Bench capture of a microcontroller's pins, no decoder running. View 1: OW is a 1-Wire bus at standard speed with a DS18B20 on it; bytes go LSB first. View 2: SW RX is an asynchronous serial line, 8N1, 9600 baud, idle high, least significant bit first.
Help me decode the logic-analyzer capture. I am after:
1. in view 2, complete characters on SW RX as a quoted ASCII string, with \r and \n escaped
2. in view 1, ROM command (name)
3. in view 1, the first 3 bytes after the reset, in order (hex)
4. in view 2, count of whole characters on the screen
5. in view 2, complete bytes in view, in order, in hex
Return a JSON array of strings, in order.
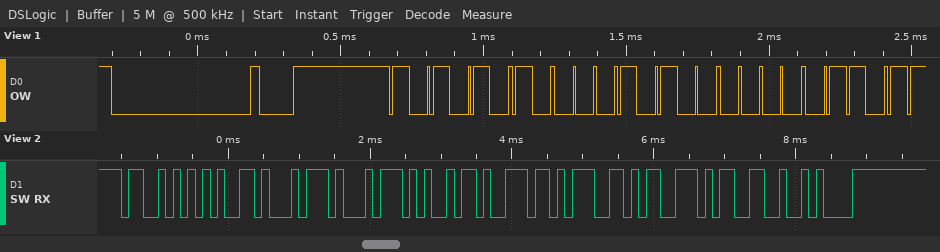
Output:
["\"Settings3\\n\"", "Match ROM", "55 28 60", "10", "53 65 74 74 69 6E 67 73 33 0A"]
